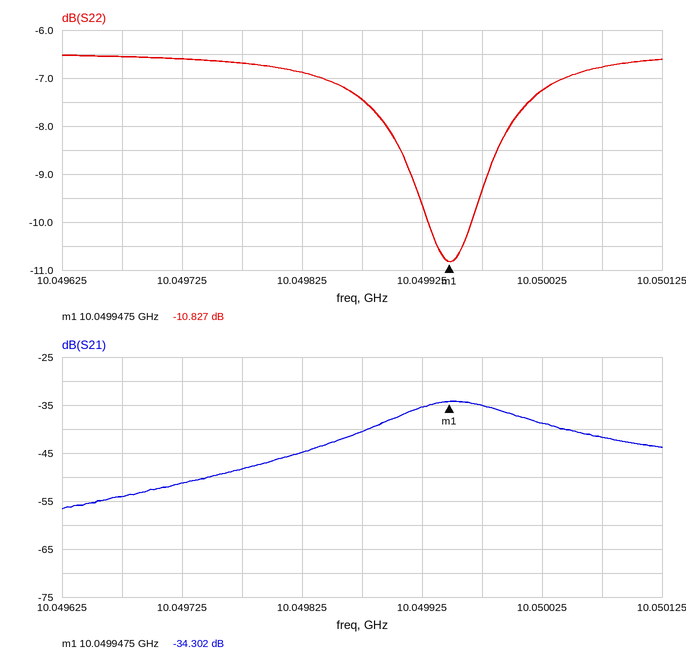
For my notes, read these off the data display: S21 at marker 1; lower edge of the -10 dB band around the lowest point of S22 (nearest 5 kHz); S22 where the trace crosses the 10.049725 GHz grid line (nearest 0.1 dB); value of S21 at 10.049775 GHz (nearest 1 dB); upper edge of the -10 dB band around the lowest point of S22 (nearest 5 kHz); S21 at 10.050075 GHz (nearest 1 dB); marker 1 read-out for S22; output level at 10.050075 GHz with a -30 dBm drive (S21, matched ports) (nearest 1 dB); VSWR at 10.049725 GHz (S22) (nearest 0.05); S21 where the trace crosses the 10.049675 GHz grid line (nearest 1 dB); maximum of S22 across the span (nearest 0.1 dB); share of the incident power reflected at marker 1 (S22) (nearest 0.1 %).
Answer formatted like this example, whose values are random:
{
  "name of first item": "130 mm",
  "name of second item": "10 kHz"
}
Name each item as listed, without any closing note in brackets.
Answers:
{
  "S21 at marker 1": "-34.302 dB",
  "lower edge of the -10 dB band around the lowest point of S22": "10.049930 GHz",
  "S22 where the trace crosses the 10.049725 GHz grid line": "-6.6 dB",
  "value of S21 at 10.049775 GHz": "-48 dB",
  "upper edge of the -10 dB band around the lowest point of S22": "10.049965 GHz",
  "S21 at 10.050075 GHz": "-42 dB",
  "marker 1 read-out for S22": "-10.827 dB",
  "output level at 10.050075 GHz with a -30 dBm drive (S21, matched ports)": "-72 dBm",
  "VSWR at 10.049725 GHz (S22)": "2.75",
  "S21 where the trace crosses the 10.049675 GHz grid line": "-54 dB",
  "maximum of S22 across the span": "-6.5 dB",
  "share of the incident power reflected at marker 1 (S22)": "8.3 %"
}
